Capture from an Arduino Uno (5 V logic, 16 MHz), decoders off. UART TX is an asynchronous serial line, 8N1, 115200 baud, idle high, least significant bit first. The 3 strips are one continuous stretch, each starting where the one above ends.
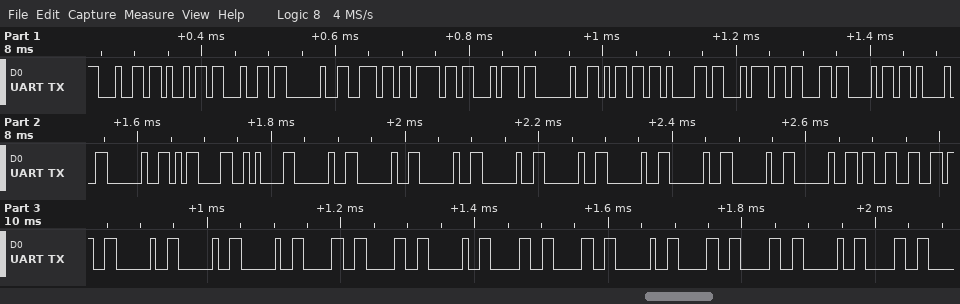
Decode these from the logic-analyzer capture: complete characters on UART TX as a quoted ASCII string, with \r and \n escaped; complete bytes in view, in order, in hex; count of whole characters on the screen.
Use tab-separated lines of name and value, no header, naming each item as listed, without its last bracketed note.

complete characters on UART TX as a quoted ASCII string, with \r and \n escaped	"did not match! \r\n         36   00 00 00 0"
complete bytes in view, in order, in hex	0x64 0x69 0x64 0x20 0x6E 0x6F 0x74 0x20 0x6D 0x61 0x74 0x63 0x68 0x21 0x20 0x0D 0x0A 0x20 0x20 0x20 0x20 0x20 0x20 0x20 0x20 0x20 0x33 0x36 0x20 0x20 0x20 0x30 0x30 0x20 0x30 0x30 0x20 0x30 0x30 0x20 0x30
count of whole characters on the screen	41
